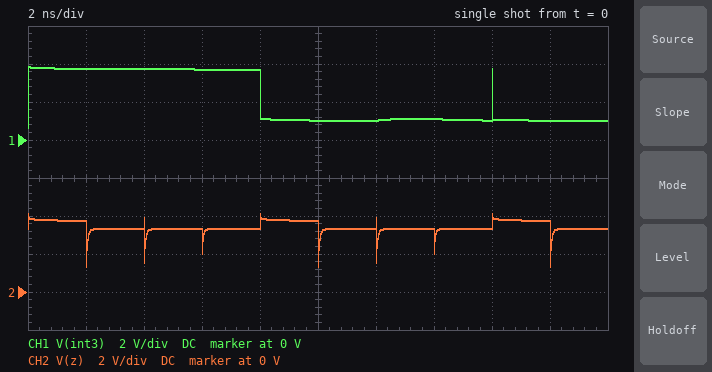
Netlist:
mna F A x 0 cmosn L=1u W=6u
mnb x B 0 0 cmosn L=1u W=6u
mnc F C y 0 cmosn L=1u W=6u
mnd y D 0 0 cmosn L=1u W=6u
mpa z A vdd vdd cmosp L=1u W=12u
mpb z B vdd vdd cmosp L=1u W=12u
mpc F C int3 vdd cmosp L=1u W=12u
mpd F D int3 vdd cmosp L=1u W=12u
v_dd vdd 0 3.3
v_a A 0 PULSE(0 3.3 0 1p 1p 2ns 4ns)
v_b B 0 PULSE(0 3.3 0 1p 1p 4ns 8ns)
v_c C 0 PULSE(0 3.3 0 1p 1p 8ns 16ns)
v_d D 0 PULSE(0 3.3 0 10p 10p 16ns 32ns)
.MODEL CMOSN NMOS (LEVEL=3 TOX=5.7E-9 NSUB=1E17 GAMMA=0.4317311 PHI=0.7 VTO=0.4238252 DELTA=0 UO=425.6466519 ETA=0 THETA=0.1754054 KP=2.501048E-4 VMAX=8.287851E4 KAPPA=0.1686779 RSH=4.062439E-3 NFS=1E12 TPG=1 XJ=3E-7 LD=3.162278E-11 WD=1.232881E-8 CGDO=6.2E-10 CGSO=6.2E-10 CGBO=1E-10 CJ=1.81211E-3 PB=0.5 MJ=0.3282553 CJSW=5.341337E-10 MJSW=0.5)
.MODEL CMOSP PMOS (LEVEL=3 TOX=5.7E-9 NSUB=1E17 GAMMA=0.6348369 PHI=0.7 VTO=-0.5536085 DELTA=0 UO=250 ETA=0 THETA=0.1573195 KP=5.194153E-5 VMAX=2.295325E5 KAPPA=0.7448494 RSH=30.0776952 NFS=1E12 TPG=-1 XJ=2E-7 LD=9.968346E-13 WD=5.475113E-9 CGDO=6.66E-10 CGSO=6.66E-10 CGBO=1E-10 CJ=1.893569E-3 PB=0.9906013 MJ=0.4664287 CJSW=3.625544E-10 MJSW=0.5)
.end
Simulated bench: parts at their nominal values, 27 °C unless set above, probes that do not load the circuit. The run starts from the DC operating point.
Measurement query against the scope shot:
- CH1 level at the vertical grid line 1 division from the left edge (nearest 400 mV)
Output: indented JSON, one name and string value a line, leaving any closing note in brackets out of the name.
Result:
{
  "CH1 level at the vertical grid line 1 division from the left edge": "3.6 V"
}
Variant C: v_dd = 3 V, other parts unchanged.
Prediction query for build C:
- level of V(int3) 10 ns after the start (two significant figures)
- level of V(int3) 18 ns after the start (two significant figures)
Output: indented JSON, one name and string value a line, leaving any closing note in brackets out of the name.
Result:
{
  "level of V(int3) 10 ns after the start": "960 mV",
  "level of V(int3) 18 ns after the start": "970 mV"
}
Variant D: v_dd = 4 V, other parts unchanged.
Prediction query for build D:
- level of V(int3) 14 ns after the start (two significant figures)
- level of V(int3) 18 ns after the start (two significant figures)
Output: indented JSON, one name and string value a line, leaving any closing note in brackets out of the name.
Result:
{
  "level of V(int3) 14 ns after the start": "1.2 V",
  "level of V(int3) 18 ns after the start": "1.1 V"
}
